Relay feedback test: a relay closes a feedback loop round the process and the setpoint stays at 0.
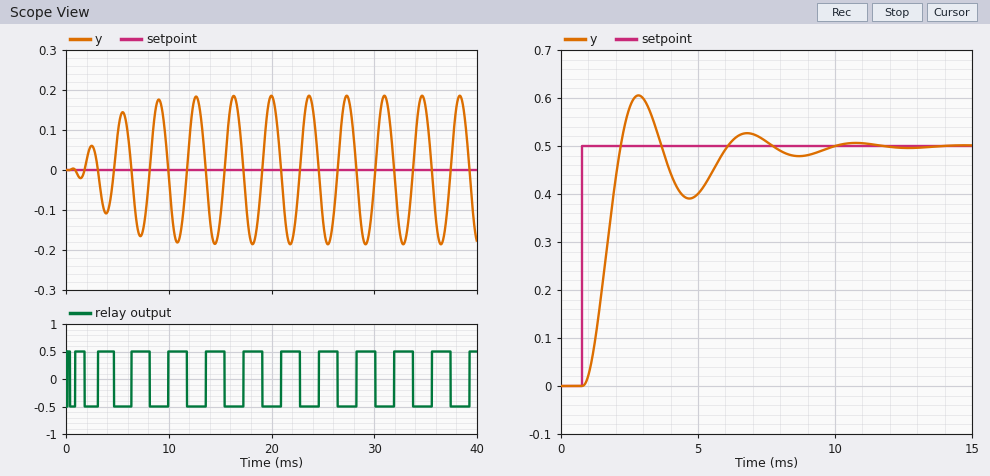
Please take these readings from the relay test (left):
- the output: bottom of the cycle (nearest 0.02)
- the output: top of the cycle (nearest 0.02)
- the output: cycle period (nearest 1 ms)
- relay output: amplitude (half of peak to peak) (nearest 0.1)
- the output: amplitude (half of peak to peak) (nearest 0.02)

-0.18
0.18
4 ms
0.5
0.18
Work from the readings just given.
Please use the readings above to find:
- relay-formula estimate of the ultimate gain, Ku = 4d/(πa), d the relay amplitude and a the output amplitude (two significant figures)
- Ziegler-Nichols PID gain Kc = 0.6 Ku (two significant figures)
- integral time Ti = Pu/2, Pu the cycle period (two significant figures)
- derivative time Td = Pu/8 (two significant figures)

3.5
2.1
2.0 ms
0.50 ms
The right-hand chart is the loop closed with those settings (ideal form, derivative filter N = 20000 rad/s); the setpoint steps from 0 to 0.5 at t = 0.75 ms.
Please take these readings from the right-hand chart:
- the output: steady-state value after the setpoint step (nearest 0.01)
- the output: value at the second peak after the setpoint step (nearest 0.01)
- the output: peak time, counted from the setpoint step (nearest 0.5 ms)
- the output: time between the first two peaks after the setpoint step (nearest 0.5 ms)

0.50
0.53
2.0 ms
4.0 ms
